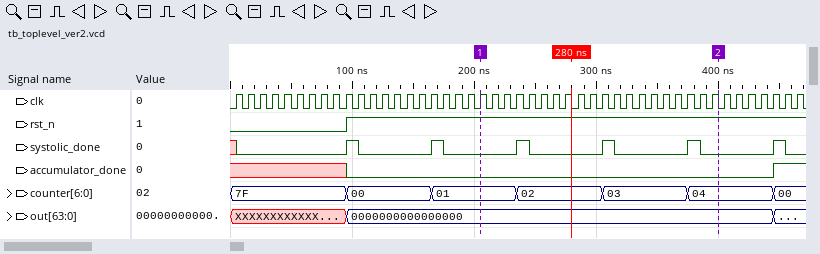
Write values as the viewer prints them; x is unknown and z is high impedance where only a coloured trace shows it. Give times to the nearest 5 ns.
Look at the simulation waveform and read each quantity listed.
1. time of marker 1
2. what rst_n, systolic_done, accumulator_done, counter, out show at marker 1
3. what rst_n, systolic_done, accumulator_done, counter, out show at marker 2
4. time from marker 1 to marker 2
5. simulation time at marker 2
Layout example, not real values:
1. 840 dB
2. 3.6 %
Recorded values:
1. 205 ns
2. rst_n=1, systolic_done=0, accumulator_done=0, counter=01, out=0000000000000000
3. rst_n=1, systolic_done=0, accumulator_done=0, counter=04, out=0000000000000000
4. 195 ns
5. 400 ns
